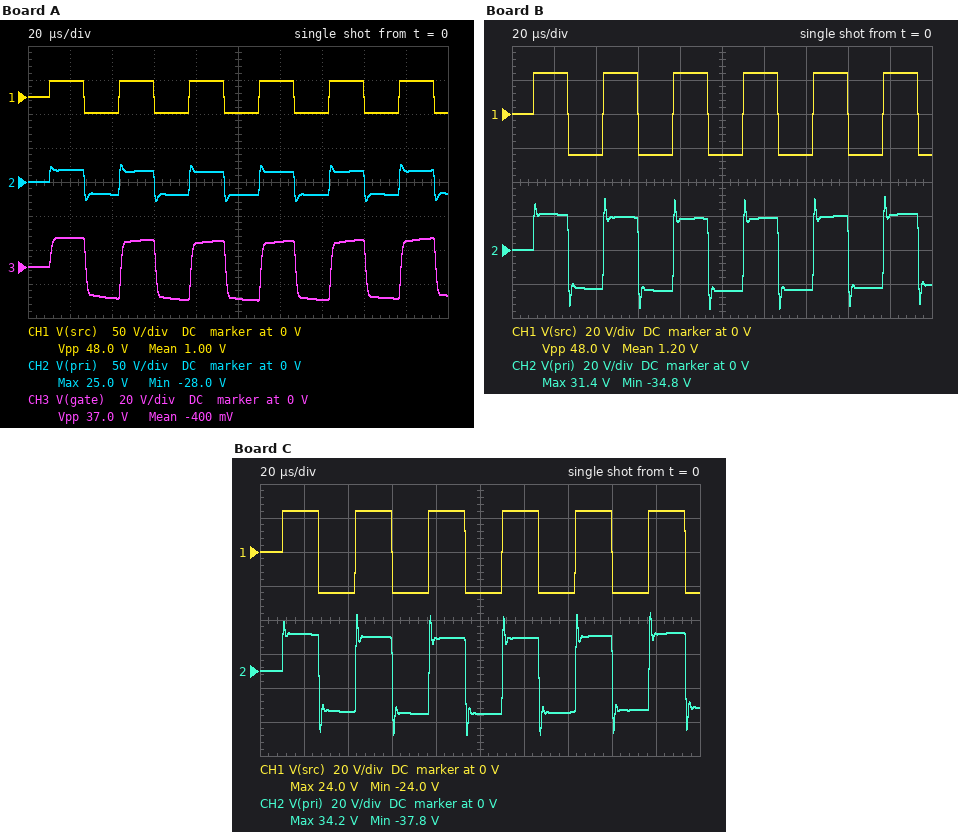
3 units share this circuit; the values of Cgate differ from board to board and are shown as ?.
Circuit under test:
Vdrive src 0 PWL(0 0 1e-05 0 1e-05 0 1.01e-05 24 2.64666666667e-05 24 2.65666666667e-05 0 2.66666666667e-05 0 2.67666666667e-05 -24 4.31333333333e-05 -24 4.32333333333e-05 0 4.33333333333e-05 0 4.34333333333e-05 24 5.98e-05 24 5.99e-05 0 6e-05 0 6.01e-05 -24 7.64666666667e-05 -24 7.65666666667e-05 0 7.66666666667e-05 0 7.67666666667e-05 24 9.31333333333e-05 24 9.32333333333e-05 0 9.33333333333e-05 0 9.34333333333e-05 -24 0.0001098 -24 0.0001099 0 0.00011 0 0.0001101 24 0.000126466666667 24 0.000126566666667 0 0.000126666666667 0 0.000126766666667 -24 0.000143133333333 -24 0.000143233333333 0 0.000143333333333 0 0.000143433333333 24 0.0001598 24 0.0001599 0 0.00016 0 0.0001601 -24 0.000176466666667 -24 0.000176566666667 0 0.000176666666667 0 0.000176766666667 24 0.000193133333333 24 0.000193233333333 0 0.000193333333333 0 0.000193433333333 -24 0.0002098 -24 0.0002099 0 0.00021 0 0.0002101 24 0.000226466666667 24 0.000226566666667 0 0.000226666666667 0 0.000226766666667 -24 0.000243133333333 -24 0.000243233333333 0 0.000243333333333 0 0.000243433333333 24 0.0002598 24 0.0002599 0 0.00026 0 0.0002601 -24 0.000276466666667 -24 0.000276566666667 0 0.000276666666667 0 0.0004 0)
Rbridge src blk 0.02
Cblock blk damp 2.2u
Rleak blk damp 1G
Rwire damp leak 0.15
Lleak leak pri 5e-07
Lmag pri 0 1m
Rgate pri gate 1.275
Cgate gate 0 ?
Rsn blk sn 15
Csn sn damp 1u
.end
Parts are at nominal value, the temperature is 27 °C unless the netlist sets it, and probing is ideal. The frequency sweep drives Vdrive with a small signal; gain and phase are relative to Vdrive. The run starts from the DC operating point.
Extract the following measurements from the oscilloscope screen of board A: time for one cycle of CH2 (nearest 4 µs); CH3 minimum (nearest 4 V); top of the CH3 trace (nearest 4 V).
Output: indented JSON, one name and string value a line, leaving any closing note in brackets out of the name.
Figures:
{
  "time for one cycle of CH2": "32 µs",
  "CH3 minimum": "-20 V",
  "top of the CH3 trace": "16 V"
}
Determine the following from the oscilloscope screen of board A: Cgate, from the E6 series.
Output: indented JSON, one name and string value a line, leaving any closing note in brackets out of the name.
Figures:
{
  "Cgate, from the E6 series": "1 µF"
}
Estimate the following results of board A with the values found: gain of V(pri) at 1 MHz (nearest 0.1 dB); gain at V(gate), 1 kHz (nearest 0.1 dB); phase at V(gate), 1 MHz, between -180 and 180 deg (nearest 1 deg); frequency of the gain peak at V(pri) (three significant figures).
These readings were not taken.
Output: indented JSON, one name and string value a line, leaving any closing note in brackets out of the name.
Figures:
{
  "gain of V(pri) at 1 MHz": "-8.1 dB",
  "gain at V(gate), 1 kHz": "-16.4 dB",
  "phase at V(gate), 1 MHz, between -180 and 180 deg": "-154 deg",
  "frequency of the gain peak at V(pri)": "2.47 kHz"
}
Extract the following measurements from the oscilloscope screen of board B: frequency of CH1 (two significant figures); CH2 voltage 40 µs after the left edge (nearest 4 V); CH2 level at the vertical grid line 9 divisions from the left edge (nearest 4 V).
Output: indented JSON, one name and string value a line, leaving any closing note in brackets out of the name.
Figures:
{
  "frequency of CH1": "30 kHz",
  "CH2 voltage 40 µs after the left edge": "-24 V",
  "CH2 level at the vertical grid line 9 divisions from the left edge": "20 V"
}
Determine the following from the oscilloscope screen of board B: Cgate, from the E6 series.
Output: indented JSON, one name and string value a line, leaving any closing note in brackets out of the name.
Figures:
{
  "Cgate, from the E6 series": "330 nF"
}
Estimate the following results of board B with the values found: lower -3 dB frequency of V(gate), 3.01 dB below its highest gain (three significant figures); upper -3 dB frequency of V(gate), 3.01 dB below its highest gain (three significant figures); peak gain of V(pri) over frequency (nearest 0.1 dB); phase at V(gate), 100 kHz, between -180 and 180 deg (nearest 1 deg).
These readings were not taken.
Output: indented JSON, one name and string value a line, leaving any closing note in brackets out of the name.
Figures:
{
  "lower -3 dB frequency of V(gate), 3.01 dB below its highest gain": "2.60 kHz",
  "upper -3 dB frequency of V(gate), 3.01 dB below its highest gain": "2.81 kHz",
  "peak gain of V(pri) over frequency": "21.3 dB",
  "phase at V(gate), 100 kHz, between -180 and 180 deg": "-16 deg"
}
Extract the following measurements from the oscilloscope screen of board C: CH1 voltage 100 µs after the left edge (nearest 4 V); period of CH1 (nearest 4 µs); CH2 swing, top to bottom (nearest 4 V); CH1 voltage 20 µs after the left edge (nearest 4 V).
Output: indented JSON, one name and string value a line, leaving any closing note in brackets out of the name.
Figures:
{
  "CH1 voltage 100 µs after the left edge": "-24 V",
  "period of CH1": "32 µs",
  "CH2 swing, top to bottom": "72 V",
  "CH1 voltage 20 µs after the left edge": "24 V"
}
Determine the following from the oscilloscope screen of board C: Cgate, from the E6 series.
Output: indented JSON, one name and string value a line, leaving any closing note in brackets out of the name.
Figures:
{
  "Cgate, from the E6 series": "220 nF"
}
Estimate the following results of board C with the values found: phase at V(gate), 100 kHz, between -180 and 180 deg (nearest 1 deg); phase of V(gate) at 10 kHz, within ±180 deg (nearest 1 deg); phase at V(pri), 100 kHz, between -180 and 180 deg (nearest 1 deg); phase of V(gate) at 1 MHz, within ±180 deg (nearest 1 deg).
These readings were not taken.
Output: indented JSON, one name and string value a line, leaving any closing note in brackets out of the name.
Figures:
{
  "phase at V(gate), 100 kHz, between -180 and 180 deg": "-11 deg",
  "phase of V(gate) at 10 kHz, within ±180 deg": "-1 deg",
  "phase at V(pri), 100 kHz, between -180 and 180 deg": "-1 deg",
  "phase of V(gate) at 1 MHz, within ±180 deg": "-148 deg"
}
